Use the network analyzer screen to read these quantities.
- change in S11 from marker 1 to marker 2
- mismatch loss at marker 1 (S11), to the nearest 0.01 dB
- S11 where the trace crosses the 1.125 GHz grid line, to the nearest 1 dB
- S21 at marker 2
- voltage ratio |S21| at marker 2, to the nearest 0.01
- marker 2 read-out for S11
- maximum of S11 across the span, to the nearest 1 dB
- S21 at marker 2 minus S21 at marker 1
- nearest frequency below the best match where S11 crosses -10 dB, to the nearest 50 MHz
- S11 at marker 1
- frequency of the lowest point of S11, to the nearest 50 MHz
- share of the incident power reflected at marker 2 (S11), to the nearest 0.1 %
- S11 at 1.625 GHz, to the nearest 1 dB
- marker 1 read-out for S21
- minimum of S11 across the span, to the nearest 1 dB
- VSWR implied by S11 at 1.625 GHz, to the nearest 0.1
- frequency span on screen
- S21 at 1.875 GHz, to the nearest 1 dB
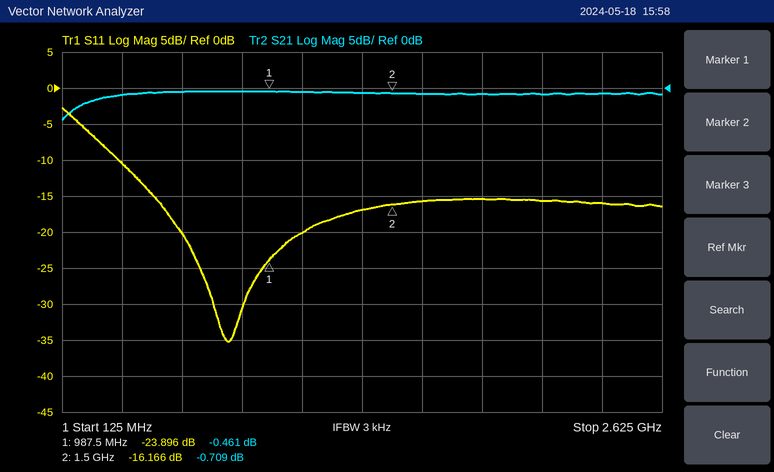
7.730 dB
0.02 dB
-20 dB
-0.709 dB
0.92
-16.166 dB
-3 dB
-0.248 dB
350 MHz
-23.896 dB
800 MHz
2.4 %
-16 dB
-0.461 dB
-35 dB
1.4
2.5 GHz
-1 dB
